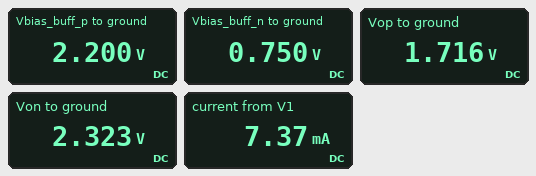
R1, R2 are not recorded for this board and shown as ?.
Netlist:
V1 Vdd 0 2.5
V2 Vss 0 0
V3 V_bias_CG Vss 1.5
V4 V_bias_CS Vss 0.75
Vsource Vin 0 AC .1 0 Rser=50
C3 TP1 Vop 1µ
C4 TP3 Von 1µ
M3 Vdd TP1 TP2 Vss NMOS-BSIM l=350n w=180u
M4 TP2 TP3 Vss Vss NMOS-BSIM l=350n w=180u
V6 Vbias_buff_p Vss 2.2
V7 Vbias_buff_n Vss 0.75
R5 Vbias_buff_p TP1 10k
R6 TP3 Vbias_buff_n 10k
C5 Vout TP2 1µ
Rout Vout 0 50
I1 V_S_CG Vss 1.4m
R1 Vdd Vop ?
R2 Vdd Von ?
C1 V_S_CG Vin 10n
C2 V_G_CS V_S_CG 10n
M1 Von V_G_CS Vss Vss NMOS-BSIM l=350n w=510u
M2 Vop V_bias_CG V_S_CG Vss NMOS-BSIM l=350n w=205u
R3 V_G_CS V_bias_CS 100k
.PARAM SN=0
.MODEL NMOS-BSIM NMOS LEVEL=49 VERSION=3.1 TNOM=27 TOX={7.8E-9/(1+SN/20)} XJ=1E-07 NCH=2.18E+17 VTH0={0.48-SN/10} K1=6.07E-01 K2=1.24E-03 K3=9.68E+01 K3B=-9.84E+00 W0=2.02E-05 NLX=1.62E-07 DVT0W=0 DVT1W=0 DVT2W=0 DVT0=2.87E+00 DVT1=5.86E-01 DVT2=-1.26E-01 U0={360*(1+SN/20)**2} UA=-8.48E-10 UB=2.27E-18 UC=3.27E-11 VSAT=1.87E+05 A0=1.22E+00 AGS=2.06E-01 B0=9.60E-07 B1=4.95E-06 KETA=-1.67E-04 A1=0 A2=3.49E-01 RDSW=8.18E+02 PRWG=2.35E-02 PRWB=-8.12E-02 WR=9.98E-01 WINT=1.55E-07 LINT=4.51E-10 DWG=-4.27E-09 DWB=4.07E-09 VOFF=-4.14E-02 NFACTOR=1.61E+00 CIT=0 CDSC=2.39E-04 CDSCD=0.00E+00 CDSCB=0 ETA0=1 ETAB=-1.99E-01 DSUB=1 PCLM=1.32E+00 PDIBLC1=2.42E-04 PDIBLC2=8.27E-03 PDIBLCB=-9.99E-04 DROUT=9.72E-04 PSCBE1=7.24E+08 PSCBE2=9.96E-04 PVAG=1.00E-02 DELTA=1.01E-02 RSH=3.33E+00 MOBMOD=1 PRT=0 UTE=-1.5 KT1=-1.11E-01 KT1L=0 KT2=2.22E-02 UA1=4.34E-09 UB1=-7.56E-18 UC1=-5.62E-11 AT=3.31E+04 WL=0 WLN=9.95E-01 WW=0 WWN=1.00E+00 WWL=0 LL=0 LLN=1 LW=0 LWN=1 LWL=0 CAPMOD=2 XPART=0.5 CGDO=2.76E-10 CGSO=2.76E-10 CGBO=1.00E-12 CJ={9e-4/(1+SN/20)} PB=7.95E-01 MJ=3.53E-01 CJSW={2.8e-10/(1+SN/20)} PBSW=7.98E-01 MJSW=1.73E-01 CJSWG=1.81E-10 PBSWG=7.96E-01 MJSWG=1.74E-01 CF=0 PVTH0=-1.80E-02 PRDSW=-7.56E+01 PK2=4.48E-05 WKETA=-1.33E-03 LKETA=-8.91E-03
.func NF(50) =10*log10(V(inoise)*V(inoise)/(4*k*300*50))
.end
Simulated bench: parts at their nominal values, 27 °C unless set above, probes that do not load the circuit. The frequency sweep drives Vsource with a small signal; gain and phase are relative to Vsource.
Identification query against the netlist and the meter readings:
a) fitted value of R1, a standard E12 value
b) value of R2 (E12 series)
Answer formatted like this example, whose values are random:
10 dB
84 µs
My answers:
560 Ω
39 Ω
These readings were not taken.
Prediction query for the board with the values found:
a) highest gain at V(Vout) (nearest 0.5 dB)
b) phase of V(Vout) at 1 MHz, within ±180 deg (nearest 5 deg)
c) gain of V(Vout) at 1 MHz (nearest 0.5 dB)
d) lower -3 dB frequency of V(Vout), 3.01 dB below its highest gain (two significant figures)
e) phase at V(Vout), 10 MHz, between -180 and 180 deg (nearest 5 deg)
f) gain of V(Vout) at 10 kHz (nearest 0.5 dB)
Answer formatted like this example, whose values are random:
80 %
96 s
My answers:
7.0 dB
10 deg
7.0 dB
140 kHz
0 deg
-16.0 dB
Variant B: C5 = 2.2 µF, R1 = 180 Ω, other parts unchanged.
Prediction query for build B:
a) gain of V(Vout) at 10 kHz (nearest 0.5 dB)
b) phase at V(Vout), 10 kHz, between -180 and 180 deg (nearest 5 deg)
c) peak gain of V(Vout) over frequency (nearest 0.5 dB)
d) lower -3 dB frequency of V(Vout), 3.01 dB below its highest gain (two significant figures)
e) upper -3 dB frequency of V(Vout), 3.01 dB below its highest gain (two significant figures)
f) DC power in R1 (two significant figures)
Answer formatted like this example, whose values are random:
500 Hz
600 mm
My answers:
-23.5 dB
90 deg
0 dB
150 kHz
2.8 GHz
350 µW
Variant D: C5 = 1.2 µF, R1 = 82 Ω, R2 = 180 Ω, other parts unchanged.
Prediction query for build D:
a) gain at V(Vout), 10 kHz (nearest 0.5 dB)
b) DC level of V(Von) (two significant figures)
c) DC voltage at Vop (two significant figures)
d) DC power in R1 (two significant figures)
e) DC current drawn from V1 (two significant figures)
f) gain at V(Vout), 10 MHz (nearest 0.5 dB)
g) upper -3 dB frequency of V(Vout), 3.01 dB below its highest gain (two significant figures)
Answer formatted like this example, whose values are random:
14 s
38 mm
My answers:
-20.0 dB
1.8 V
2.4 V
160 µW
6.9 mA
3.5 dB
1.4 GHz
